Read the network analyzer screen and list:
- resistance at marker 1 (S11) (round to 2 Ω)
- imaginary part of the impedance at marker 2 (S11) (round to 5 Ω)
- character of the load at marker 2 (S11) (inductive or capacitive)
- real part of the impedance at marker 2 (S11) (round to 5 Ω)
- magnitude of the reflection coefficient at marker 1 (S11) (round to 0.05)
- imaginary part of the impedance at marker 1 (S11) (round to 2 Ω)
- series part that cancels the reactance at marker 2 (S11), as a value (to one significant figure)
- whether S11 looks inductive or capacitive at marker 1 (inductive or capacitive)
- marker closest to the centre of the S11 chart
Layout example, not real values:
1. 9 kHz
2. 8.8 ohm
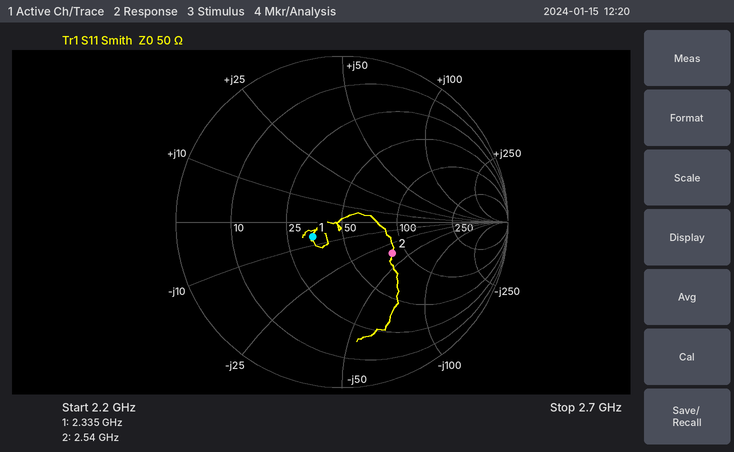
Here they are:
1. 34 Ω
2. -35 Ω
3. capacitive
4. 85 Ω
5. 0.20
6. -6 Ω
7. 2 nH
8. capacitive
9. marker 1
